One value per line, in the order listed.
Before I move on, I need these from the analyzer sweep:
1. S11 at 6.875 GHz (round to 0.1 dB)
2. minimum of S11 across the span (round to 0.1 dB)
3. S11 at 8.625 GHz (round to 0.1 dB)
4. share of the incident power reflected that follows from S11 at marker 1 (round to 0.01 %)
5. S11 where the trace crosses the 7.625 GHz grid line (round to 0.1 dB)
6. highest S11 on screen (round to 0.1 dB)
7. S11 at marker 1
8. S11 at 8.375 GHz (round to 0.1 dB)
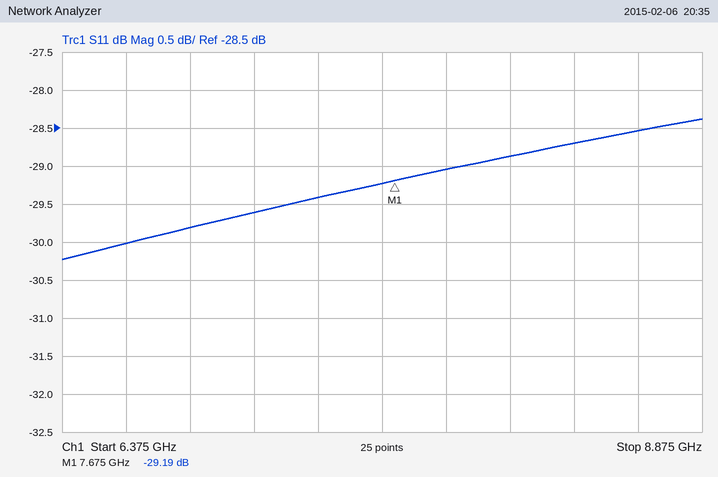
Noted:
-29.8 dB
-30.2 dB
-28.5 dB
0.12 %
-29.2 dB
-28.4 dB
-29.19 dB
-28.7 dB
